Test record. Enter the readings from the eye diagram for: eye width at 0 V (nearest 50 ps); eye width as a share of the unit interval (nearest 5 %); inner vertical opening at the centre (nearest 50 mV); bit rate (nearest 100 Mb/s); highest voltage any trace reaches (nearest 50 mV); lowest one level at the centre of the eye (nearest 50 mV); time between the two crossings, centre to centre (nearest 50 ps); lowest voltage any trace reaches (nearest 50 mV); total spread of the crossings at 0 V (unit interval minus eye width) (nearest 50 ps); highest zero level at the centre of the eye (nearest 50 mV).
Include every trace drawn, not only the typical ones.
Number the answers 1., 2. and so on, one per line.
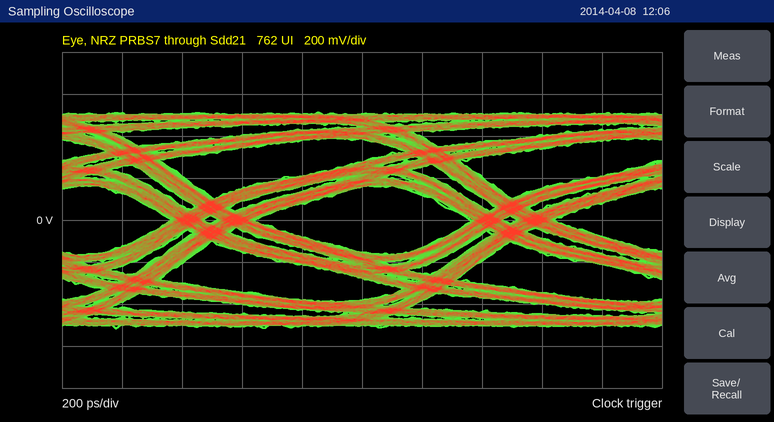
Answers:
1. 700 ps
2. 70 %
3. 300 mV
4. 1.0 Gb/s
5. 500 mV
6. 150 mV
7. 1.00 ns
8. -500 mV
9. 300 ps
10. -150 mV
